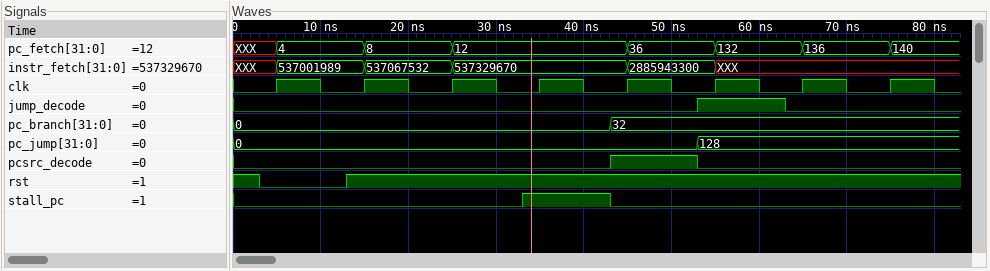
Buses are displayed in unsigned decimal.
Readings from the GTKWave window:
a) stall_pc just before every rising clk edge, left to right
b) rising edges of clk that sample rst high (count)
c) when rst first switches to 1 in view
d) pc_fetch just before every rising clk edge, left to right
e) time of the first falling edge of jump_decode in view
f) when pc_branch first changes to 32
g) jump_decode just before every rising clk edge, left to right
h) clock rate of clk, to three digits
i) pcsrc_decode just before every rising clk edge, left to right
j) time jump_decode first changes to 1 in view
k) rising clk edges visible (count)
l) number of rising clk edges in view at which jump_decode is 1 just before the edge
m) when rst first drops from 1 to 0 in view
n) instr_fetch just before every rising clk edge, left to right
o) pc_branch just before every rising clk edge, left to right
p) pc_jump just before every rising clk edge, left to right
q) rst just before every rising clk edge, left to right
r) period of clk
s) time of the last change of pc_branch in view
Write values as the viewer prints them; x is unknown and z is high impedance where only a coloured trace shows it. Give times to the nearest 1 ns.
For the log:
0 0 0 1 0 0 0 0
7
13 ns
XXX, 4, 8, 12, 12, 36, 132, 136
63 ns
43 ns
0 0 0 0 0 1 0 0
100 MHz
0 0 0 0 1 0 0 0
53 ns
8
1
3 ns
XXX, 537001989, 537067532, 537329670, 537329670, 2885943300, XXX, XXX
0, 0, 0, 0, 32, 32, 32, 32
0, 0, 0, 0, 0, 128, 128, 128
0 1 1 1 1 1 1 1
10 ns
43 ns
